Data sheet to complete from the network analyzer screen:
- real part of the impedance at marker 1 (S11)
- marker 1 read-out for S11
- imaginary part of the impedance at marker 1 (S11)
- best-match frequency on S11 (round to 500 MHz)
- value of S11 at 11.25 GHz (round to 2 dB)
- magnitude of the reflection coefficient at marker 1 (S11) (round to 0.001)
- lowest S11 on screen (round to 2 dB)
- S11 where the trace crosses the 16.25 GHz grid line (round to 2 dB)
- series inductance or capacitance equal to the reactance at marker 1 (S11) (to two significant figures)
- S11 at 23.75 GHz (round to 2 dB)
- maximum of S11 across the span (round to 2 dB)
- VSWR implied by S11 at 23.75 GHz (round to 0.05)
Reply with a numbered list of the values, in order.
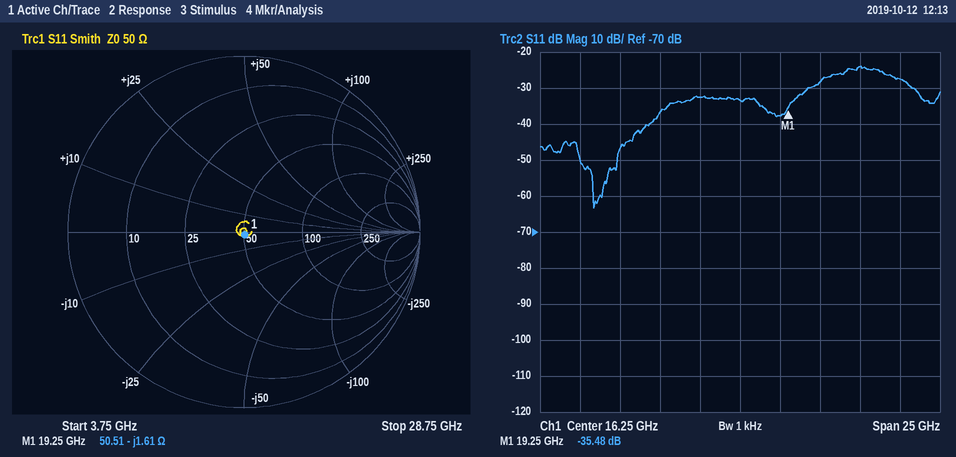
1. 50.51 Ω
2. -35.48 dB
3. -1.61 Ω
4. 7.0 GHz
5. -36 dB
6. 0.017
7. -64 dB
8. -34 dB
9. 5.1 pF
10. -24 dB
11. -24 dB
12. 1.15
